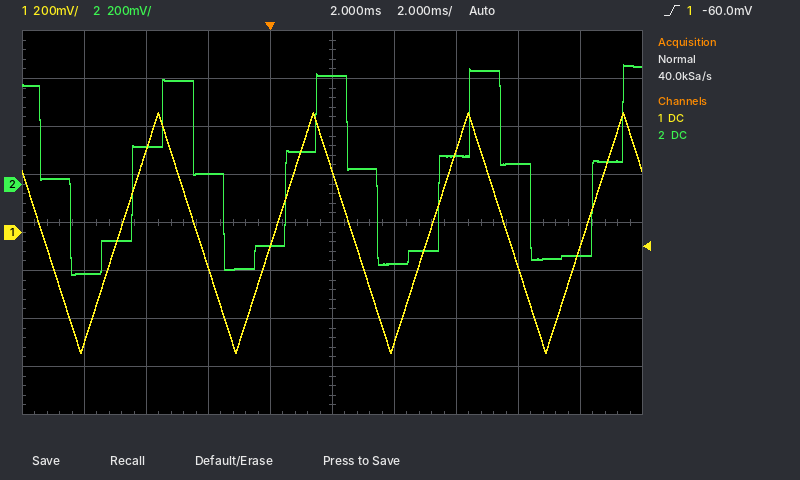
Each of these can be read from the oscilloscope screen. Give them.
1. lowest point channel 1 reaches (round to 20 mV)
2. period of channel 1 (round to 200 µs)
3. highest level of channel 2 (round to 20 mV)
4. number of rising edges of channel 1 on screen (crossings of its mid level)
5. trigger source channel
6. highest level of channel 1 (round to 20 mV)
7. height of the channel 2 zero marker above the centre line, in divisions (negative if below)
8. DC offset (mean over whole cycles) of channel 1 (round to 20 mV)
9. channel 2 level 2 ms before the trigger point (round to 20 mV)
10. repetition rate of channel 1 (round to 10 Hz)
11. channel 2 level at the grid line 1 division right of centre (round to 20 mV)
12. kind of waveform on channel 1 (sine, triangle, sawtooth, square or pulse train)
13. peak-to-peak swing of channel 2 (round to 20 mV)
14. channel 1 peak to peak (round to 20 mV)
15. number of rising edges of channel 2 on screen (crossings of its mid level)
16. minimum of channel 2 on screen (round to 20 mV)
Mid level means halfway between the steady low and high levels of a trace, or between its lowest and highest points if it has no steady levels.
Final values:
-500 mV
5.0 ms
500 mV
4
channel 1
500 mV
+0.8 div
0 mV
40 mV
200 Hz
-340 mV
triangle
880 mV
1.00 V
4
-380 mV
